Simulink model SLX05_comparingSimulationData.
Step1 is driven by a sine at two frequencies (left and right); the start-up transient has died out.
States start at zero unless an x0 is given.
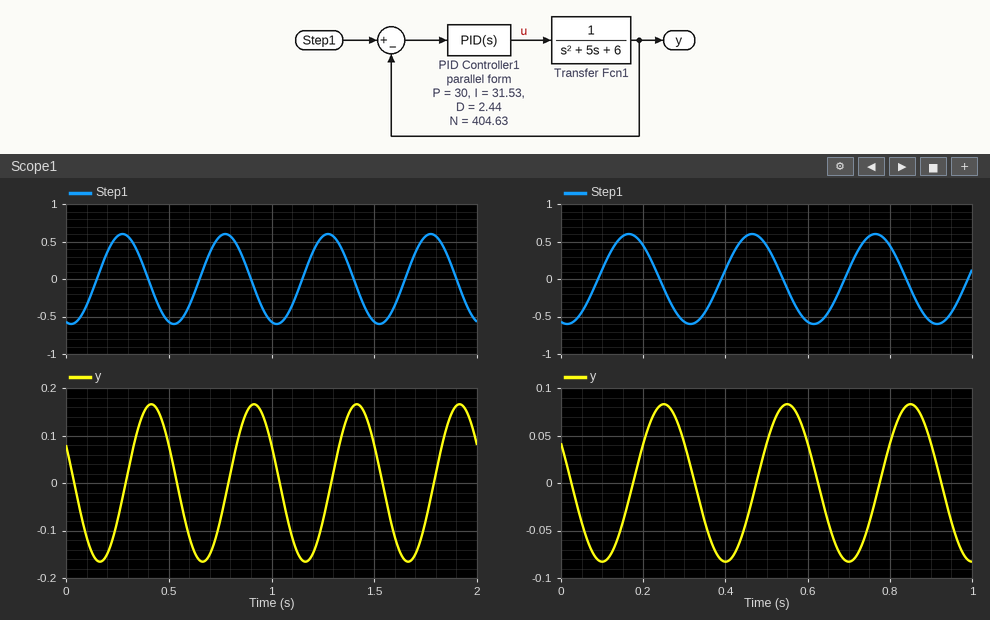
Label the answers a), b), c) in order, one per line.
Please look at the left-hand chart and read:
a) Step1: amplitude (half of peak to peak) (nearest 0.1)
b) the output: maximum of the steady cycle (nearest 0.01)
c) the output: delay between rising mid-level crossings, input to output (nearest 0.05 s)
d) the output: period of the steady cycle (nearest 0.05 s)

a) 0.6
b) 0.17
c) 0.15 s
d) 0.50 s
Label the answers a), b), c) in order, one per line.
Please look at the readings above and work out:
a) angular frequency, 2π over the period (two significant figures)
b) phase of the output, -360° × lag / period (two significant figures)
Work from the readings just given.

a) 13 rad/s
b) -110°
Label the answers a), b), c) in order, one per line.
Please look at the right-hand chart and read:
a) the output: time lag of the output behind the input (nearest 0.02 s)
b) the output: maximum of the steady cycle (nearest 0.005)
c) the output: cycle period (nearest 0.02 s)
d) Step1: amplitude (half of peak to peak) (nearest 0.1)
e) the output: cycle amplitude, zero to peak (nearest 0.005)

a) 0.08 s
b) 0.085
c) 0.30 s
d) 0.6
e) 0.085
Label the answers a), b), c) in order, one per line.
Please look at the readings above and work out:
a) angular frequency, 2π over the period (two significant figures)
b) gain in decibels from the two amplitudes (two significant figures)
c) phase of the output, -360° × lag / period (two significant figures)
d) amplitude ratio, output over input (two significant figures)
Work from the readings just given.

a) 21 rad/s
b) -17 dB
c) -96°
d) 0.14
